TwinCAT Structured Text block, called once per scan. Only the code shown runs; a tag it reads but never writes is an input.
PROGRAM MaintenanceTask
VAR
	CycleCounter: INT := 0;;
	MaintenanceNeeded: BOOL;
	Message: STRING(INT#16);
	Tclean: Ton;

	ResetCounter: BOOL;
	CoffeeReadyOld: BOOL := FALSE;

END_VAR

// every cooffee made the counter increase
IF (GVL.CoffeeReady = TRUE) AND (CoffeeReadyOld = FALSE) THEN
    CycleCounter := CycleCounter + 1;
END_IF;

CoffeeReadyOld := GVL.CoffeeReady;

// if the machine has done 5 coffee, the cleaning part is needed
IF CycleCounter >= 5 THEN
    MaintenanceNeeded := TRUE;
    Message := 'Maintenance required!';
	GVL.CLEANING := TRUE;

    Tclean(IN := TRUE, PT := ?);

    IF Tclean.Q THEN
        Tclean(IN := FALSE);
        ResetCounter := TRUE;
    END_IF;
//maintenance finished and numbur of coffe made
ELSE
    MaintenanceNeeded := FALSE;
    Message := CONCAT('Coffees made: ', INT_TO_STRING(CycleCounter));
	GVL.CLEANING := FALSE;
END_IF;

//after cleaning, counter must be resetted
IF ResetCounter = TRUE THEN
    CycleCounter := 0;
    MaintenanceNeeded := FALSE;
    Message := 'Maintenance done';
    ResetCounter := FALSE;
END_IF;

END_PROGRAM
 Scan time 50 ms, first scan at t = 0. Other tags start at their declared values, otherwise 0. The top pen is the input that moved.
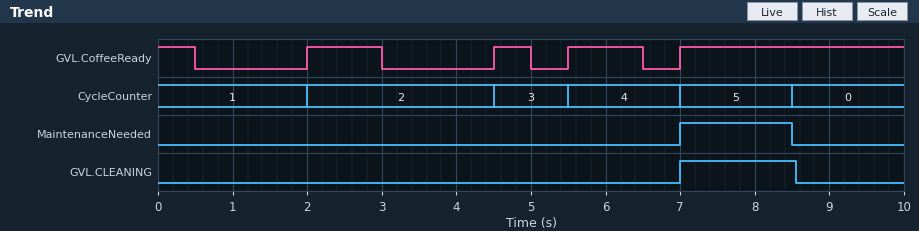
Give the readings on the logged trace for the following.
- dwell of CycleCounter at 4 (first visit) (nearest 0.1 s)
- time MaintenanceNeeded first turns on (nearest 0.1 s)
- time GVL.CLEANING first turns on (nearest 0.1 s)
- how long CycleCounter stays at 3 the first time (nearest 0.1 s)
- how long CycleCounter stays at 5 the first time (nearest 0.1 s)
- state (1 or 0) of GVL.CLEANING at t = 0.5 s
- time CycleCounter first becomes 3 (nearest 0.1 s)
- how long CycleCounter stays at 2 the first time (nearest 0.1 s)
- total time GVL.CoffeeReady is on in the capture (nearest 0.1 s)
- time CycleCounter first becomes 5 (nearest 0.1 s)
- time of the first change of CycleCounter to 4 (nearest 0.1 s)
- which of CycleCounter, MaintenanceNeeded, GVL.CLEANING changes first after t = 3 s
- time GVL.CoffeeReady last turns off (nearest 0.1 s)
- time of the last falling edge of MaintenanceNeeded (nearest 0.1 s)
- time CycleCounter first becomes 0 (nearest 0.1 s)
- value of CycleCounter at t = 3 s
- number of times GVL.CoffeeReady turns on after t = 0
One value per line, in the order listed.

1.5 s
7.0 s
7.0 s
1.0 s
1.5 s
0
4.5 s
2.5 s
6.0 s
7.0 s
5.5 s
CycleCounter
6.5 s
8.5 s
8.5 s
2
4
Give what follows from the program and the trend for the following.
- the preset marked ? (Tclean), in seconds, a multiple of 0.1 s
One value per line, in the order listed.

1.5 s
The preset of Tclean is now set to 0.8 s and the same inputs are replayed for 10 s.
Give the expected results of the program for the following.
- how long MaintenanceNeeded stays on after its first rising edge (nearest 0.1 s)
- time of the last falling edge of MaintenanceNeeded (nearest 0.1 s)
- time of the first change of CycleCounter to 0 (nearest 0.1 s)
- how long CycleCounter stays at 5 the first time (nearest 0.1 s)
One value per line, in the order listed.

0.8 s
7.8 s
7.8 s
0.8 s
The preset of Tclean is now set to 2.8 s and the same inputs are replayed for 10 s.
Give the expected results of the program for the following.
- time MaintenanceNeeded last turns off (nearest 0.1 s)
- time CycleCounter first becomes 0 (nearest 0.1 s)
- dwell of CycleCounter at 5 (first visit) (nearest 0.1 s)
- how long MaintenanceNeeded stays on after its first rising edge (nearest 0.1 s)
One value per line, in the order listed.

9.8 s
9.8 s
2.8 s
2.8 s
